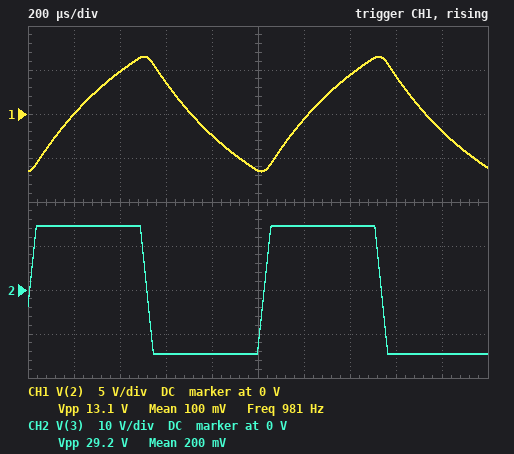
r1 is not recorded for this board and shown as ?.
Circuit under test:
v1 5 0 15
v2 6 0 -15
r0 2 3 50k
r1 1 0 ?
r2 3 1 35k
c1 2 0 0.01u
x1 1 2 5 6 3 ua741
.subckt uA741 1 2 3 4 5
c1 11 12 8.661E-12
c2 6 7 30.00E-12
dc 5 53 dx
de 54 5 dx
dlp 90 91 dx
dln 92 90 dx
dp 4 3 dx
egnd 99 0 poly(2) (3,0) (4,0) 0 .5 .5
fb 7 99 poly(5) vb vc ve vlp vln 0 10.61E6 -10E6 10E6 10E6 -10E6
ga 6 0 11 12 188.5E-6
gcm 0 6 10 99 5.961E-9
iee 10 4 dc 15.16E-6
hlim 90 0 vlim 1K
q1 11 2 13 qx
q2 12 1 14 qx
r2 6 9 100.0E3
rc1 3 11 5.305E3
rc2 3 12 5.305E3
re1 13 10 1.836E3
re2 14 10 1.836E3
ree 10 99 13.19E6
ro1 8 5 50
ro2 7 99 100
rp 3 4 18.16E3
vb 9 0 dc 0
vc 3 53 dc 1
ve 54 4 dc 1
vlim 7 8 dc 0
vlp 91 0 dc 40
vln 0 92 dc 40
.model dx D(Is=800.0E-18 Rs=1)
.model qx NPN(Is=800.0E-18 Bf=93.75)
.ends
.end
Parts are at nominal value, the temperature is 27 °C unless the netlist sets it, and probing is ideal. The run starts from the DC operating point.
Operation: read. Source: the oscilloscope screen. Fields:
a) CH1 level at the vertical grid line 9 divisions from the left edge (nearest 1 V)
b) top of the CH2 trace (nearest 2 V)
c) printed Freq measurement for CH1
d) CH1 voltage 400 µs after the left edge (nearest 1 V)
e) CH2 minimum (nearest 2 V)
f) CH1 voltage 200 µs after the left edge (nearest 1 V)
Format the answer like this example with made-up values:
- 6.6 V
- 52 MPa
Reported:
- -2 V
- 14 V
- 981 Hz
- 5 V
- -14 V
- 0 V
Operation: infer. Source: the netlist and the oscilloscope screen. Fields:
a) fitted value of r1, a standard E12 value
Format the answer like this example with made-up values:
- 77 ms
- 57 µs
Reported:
- 27 kΩ
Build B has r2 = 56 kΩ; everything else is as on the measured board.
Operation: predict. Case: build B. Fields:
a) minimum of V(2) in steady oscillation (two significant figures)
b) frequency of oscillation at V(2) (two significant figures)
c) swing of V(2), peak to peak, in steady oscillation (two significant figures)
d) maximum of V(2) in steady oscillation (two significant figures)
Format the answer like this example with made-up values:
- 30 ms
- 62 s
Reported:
- -5.0 V
- 1.3 kHz
- 10 V
- 5.0 V
